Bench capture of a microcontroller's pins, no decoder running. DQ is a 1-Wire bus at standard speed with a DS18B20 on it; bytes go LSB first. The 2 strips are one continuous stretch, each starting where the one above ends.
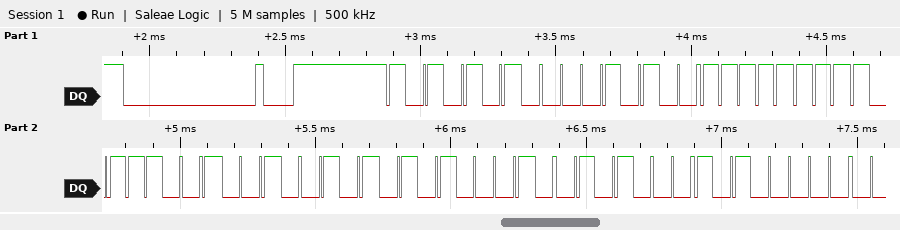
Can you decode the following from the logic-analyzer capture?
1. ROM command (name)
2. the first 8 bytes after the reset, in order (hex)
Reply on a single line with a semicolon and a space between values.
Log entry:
Match ROM; 55 28 FF 9D A4 8A 14 05
